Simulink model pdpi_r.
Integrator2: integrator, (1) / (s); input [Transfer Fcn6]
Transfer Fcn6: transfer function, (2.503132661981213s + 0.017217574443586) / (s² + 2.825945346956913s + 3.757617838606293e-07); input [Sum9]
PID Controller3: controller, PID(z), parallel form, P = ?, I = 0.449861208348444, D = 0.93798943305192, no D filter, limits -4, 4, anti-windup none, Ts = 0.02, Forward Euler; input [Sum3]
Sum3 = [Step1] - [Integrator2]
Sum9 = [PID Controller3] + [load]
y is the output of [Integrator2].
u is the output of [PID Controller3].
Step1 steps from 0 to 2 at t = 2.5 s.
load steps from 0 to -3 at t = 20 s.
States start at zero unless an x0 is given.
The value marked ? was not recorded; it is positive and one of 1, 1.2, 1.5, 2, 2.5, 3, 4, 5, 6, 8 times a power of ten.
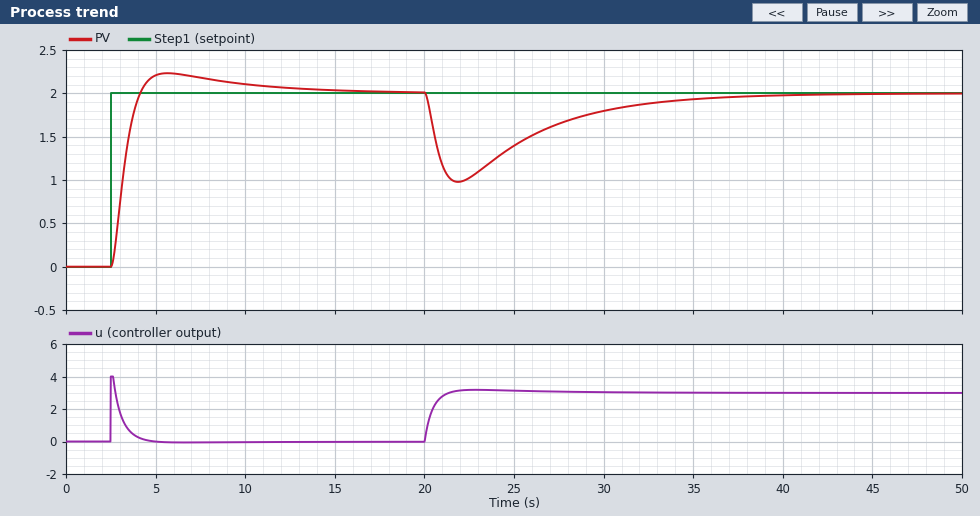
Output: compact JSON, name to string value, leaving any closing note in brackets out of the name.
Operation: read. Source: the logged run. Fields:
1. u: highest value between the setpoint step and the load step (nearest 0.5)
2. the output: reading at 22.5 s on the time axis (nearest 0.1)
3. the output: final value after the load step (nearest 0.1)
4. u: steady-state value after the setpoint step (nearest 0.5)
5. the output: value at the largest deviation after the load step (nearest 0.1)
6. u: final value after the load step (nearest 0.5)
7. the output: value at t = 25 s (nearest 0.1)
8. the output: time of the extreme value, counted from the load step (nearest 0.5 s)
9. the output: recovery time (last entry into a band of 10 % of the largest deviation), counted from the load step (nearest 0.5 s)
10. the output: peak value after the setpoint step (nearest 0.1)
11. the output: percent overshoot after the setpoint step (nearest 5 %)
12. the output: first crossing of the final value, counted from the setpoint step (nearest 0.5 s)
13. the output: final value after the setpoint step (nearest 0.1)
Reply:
{"u: highest value between the setpoint step and the load step": "4.0", "the output: reading at 22.5 s on the time axis": "1.0", "the output: final value after the load step": "2.0", "u: steady-state value after the setpoint step": "0.0", "the output: value at the largest deviation after the load step": "1.0", "u: final value after the load step": "3.0", "the output: value at t = 25 s": "1.4", "the output: time of the extreme value, counted from the load step": "2.0 s", "the output: recovery time (last entry into a band of 10 % of the largest deviation), counted from the load step": "13.0 s", "the output: peak value after the setpoint step": "2.2", "the output: percent overshoot after the setpoint step": "10 %", "the output: first crossing of the final value, counted from the setpoint step": "1.5 s", "the output: final value after the setpoint step": "2.0"}
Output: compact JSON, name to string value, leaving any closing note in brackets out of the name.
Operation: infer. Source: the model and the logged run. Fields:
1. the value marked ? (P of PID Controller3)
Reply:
{"the value marked ?": "2.5"}
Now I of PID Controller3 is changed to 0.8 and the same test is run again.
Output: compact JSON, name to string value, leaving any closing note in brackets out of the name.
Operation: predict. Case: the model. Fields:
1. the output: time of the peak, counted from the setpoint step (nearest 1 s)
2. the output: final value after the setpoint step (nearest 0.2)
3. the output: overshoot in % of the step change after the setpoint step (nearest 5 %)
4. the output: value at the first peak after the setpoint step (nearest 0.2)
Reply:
{"the output: time of the peak, counted from the setpoint step": "3 s", "the output: final value after the setpoint step": "2.0", "the output: overshoot in % of the step change after the setpoint step": "20 %", "the output: value at the first peak after the setpoint step": "2.4"}
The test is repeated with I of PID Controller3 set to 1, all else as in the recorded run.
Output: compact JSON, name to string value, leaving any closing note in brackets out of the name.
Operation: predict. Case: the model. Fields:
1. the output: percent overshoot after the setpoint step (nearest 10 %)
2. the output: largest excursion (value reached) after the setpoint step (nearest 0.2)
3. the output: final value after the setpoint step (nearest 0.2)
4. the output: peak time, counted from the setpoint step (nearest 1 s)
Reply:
{"the output: percent overshoot after the setpoint step": "20 %", "the output: largest excursion (value reached) after the setpoint step": "2.4", "the output: final value after the setpoint step": "2.0", "the output: peak time, counted from the setpoint step": "3 s"}
